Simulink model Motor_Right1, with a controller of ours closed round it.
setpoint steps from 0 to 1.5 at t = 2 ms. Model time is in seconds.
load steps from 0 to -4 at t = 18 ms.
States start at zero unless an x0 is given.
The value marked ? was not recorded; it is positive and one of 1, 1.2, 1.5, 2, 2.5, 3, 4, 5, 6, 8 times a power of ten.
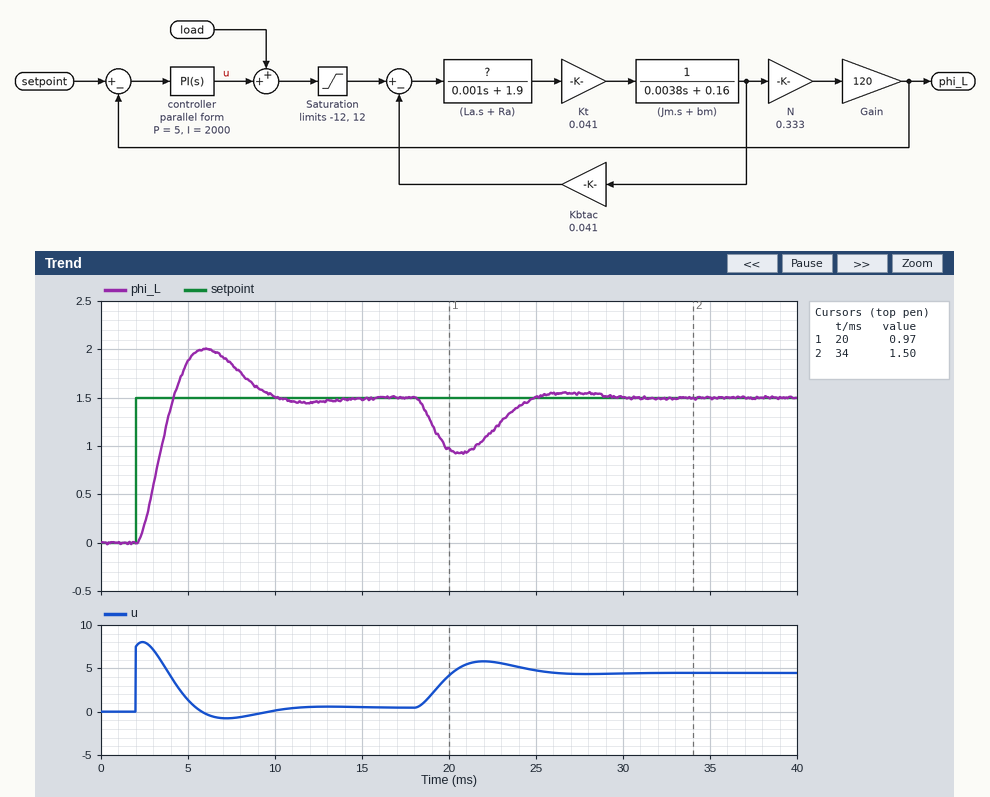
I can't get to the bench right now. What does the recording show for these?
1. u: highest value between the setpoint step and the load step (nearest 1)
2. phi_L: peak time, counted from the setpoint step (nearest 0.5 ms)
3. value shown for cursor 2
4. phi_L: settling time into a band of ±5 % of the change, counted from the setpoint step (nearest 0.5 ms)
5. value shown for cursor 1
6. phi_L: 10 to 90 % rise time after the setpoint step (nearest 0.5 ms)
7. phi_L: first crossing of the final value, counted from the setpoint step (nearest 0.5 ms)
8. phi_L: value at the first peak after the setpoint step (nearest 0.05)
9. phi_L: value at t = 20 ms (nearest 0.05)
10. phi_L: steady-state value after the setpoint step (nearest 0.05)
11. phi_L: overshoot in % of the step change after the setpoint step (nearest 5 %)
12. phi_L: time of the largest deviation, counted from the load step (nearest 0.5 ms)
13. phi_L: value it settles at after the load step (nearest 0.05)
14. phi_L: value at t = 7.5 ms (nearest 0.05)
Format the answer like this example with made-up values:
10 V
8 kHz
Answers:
8
4.0 ms
1.50
7.5 ms
0.97
1.5 ms
2.0 ms
2.00
0.95
1.50
35 %
2.5 ms
1.50
1.85
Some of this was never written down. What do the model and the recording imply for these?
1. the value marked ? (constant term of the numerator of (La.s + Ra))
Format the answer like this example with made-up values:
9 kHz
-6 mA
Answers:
0.6
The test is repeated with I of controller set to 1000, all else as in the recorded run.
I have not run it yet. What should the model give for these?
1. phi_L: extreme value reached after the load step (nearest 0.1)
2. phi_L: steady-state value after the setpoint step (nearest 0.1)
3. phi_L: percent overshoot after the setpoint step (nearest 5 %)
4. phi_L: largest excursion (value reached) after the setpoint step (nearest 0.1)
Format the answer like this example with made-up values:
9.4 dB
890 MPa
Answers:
0.9
1.5
20 %
1.8
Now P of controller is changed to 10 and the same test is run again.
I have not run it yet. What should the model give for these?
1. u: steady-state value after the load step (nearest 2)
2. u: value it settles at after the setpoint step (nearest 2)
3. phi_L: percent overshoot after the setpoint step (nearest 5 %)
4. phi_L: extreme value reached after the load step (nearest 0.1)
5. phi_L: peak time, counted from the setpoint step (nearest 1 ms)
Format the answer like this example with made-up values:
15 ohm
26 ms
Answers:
4
0
25 %
1.1
3 ms
